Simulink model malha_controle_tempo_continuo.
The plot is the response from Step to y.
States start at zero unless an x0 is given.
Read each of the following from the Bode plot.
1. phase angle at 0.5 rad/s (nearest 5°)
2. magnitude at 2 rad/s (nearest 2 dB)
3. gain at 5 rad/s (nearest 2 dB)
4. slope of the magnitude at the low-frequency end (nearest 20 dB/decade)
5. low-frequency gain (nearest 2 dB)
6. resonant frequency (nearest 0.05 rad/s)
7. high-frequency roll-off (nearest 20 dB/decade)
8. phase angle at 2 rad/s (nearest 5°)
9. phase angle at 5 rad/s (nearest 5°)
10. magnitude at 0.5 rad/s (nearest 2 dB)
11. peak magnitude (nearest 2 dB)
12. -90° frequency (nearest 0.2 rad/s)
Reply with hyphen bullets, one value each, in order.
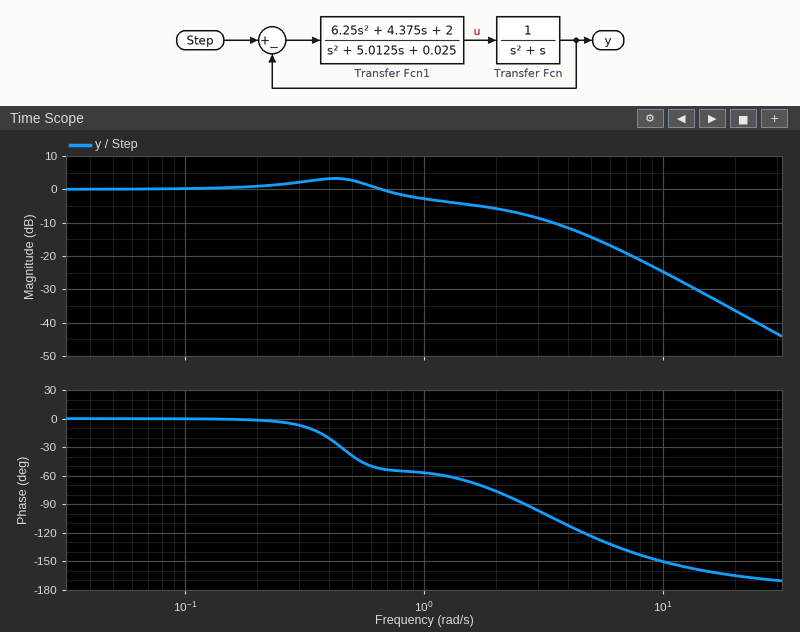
- -40°
- -6 dB
- -14 dB
- 0 dB/decade
- 0 dB
- 0.40 rad/s
- -40 dB/decade
- -75°
- -125°
- 2 dB
- 4 dB
- 2.6 rad/s
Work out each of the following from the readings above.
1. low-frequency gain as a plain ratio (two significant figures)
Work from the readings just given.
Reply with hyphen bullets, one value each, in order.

- 1.0
